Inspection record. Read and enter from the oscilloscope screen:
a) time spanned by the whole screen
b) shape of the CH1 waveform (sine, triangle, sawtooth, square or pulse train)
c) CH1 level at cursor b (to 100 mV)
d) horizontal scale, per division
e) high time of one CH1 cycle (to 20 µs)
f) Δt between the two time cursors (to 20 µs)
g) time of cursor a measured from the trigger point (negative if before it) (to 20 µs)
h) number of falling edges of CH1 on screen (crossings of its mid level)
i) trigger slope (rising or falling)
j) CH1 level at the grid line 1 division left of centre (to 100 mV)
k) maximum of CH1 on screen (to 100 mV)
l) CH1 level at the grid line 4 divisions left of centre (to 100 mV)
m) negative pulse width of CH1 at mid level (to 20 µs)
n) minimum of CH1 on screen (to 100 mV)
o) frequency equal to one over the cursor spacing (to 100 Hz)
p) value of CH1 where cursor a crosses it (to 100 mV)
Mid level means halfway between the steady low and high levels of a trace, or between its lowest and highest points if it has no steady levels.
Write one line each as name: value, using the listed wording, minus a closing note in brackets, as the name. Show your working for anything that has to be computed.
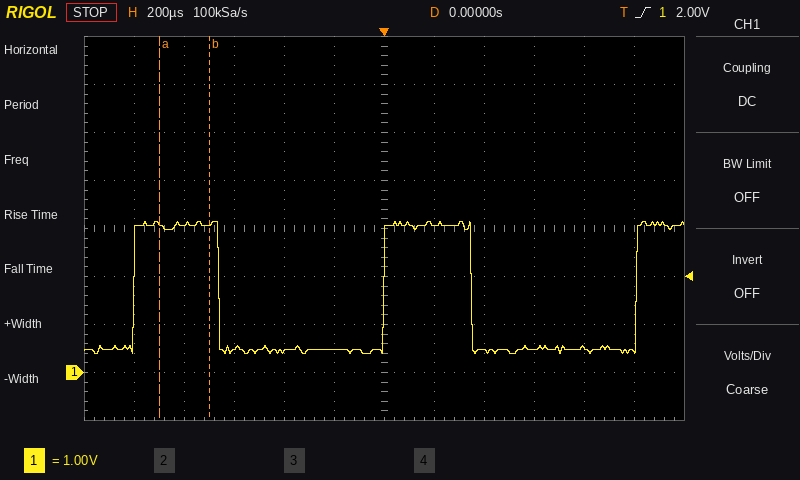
time spanned by the whole screen: 2.4 ms
shape of the CH1 waveform: pulse train
CH1 level at cursor b: 3.1 V
horizontal scale, per division: 200 µs
high time of one CH1 cycle: 340 µs
Δt between the two time cursors: 200 µs
time of cursor a measured from the trigger point (negative if before it): -900 µs
number of falling edges of CH1 on screen: 2
trigger slope: rising
CH1 level at the grid line 1 division left of centre: 500 mV
maximum of CH1 on screen: 3.1 V
CH1 level at the grid line 4 divisions left of centre: 3.1 V
negative pulse width of CH1 at mid level: 660 µs
minimum of CH1 on screen: 400 mV
frequency equal to one over the cursor spacing: 1 / 200 µs ≈ 5.0 kHz
value of CH1 where cursor a crosses it: 3.1 V
